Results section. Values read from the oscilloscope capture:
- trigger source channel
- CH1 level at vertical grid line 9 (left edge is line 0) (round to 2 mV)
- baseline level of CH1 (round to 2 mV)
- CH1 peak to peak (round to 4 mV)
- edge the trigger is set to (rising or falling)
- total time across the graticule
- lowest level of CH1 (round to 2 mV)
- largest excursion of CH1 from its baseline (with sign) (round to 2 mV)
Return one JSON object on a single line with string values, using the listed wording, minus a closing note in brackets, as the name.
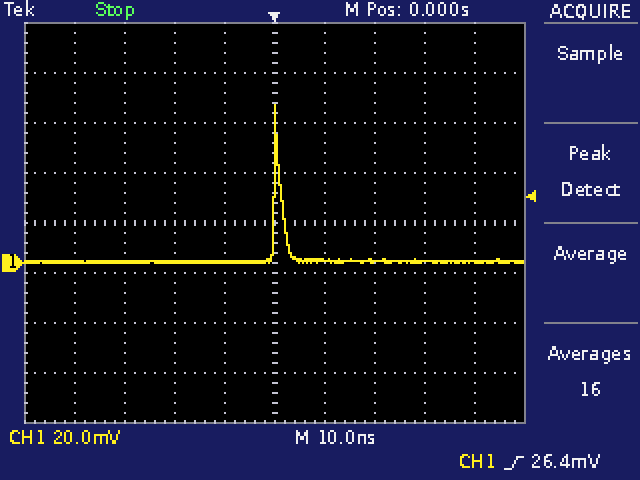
{"trigger source channel": "CH1", "CH1 level at vertical grid line 9 (left edge is line 0)": "0 mV", "baseline level of CH1": "0 mV", "CH1 peak to peak": "64 mV", "edge the trigger is set to": "rising", "total time across the graticule": "100 ns", "lowest level of CH1": "0 mV", "largest excursion of CH1 from its baseline (with sign)": "+62 mV"}
